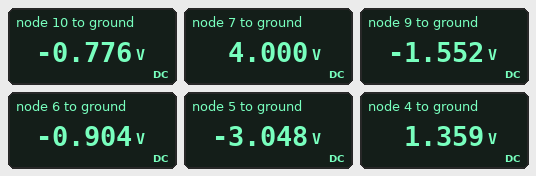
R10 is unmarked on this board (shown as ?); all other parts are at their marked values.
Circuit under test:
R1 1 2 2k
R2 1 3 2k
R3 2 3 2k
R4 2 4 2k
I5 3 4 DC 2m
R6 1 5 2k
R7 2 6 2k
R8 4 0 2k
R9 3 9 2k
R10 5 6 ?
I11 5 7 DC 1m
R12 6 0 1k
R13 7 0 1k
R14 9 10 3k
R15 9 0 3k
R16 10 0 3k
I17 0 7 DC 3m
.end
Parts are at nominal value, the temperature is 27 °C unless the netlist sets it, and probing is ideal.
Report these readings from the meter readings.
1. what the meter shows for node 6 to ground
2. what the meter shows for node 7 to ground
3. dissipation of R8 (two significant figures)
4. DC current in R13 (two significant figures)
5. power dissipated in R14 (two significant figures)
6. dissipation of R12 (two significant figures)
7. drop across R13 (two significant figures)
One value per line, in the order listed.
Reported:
-0.904 V
4.000 V
920 µW
4.0 mA
200 µW
820 µW
4.0 V
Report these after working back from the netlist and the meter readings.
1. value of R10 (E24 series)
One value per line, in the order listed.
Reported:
3 kΩ
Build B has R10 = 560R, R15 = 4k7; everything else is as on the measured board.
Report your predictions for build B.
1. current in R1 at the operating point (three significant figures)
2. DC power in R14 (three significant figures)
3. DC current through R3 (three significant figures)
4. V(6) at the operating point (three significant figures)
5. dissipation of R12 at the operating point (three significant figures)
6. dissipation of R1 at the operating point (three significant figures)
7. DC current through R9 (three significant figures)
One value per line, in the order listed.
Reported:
396 µA
224 µW
887 µA
-1.10 V
1.21 mW
314 µW
622 µA
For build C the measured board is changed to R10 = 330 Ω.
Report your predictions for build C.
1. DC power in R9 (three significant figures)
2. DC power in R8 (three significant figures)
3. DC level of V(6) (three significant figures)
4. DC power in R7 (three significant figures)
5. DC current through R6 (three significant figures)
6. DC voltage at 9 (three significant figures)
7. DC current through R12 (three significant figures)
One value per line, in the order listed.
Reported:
898 µW
1.13 mW
-1.08 V
4.09 µW
127 µA
-1.34 V
1.08 mA
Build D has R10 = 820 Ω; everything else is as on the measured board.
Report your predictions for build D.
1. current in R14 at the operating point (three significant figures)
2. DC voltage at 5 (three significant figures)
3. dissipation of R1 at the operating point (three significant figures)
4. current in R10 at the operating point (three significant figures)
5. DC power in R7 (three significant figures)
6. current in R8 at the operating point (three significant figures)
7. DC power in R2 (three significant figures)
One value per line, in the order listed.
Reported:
233 µA
-1.87 V
355 µW
1.02 mA
516 nW
733 µA
388 µW
